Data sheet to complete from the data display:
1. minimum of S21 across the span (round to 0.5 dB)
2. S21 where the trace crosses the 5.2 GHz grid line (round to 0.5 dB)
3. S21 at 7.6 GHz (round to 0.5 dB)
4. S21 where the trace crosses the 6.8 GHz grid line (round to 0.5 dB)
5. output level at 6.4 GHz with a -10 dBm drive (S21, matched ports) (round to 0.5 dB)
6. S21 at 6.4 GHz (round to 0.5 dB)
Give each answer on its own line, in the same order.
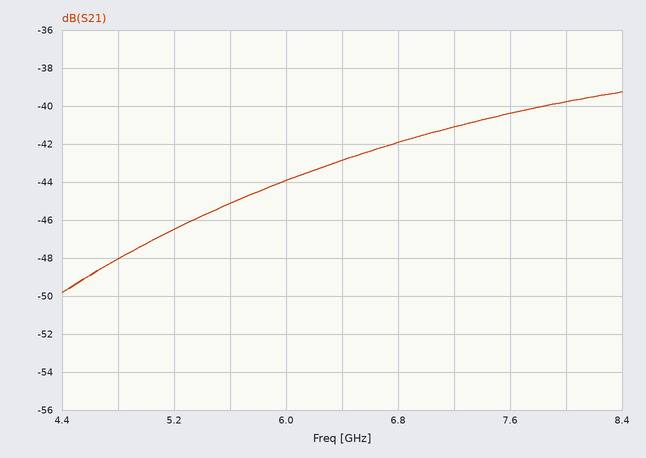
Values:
-50.0 dB
-46.5 dB
-40.5 dB
-42.0 dB
-53.0 dBm
-43.0 dB
